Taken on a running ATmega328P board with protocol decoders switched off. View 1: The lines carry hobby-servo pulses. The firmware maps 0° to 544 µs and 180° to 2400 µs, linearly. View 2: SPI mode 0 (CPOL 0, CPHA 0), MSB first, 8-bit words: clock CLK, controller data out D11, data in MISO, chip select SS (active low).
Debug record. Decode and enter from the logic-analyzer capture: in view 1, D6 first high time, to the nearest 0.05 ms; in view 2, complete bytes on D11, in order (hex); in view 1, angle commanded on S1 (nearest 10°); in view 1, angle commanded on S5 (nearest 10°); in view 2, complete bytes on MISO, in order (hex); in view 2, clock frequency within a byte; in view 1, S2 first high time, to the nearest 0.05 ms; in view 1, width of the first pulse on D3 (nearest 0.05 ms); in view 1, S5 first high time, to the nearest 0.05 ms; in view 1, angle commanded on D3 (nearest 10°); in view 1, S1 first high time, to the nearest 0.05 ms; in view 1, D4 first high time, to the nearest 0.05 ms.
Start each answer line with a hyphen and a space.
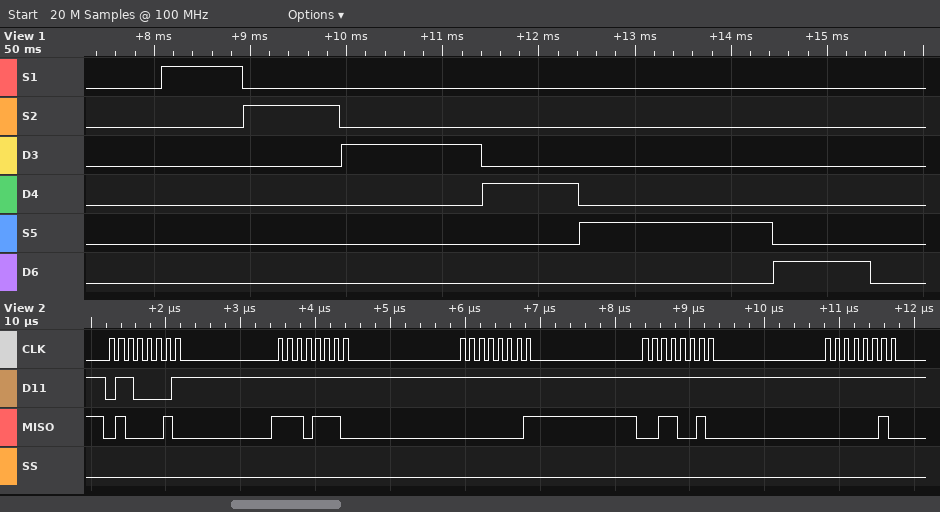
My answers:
- 1.00 ms
- 0x61 0xFF 0xFF 0xFF 0xFF
- 30°
- 140°
- 0x42 0xEE 0x01 0x32 0x02
- 8 MHz
- 1.00 ms
- 1.45 ms
- 2.00 ms
- 90°
- 0.85 ms
- 1.00 ms
